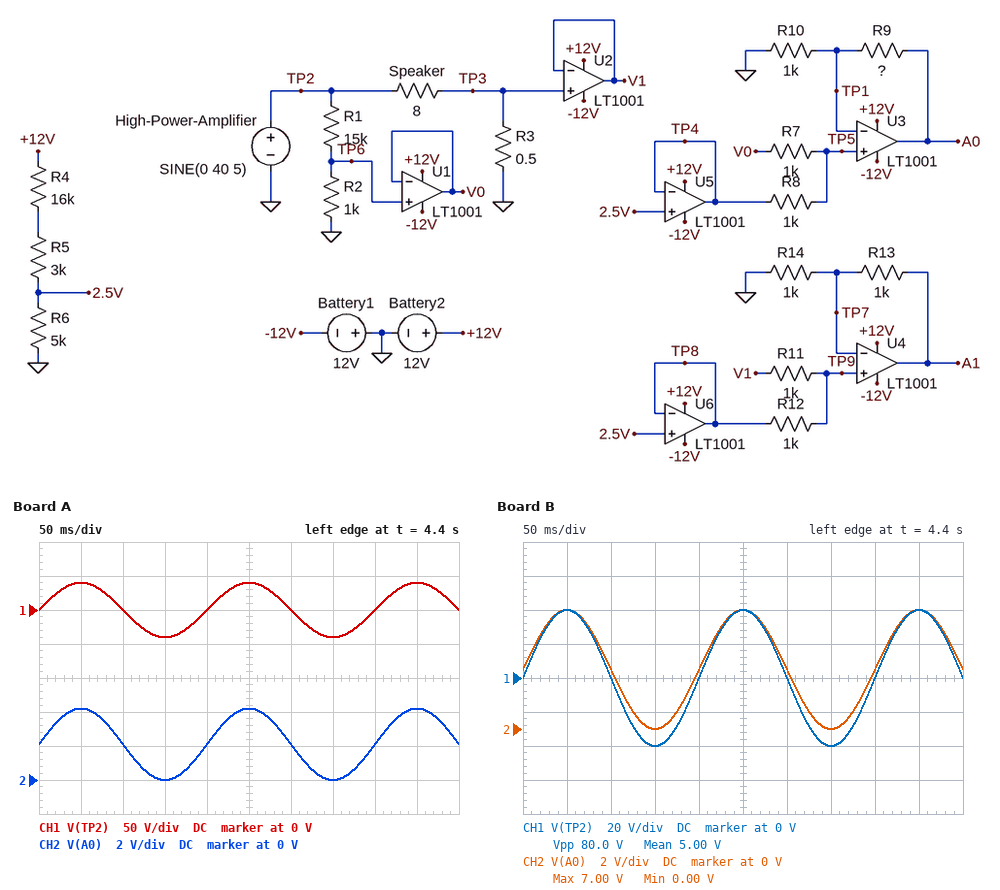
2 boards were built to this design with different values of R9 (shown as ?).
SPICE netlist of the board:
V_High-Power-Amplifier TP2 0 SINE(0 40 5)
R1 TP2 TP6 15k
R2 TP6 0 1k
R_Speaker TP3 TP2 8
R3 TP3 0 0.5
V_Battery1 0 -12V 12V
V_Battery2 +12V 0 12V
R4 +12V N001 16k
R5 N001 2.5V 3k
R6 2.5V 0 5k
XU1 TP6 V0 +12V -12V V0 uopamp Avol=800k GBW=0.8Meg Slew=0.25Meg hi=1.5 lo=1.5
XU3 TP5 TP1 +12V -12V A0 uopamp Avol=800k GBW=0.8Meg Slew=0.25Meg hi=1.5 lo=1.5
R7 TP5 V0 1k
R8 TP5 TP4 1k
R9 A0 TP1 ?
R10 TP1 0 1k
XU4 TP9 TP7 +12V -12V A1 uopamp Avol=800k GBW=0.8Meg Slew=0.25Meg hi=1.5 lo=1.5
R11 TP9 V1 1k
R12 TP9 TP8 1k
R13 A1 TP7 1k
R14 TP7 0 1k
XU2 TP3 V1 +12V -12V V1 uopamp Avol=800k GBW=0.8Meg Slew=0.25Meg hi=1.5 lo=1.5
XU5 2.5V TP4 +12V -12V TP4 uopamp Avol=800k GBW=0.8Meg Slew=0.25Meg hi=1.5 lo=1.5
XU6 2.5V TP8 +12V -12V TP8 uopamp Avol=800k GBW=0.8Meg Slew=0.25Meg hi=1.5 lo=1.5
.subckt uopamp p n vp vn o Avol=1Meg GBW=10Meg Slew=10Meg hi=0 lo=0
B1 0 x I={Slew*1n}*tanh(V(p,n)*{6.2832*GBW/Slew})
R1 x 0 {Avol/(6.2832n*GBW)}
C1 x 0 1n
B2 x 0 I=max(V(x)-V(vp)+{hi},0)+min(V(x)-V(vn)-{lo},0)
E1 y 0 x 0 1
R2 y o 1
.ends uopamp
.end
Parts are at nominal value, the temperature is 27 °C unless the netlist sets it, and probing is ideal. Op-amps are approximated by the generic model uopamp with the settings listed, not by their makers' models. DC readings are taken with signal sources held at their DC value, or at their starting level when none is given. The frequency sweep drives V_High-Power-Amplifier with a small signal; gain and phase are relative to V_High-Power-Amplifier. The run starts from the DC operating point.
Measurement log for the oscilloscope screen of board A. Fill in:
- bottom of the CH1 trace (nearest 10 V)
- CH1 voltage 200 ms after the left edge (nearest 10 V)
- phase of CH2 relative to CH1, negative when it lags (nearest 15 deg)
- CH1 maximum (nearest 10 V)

-40 V
0 V
0 deg
40 V
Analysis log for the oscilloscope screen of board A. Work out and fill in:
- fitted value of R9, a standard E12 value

680 Ω
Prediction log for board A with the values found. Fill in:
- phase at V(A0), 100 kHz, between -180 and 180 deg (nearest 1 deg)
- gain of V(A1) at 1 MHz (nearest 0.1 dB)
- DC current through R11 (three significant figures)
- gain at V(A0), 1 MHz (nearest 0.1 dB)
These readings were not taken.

-19 deg
-37.3 dB
1.25 mA
-37.0 dB
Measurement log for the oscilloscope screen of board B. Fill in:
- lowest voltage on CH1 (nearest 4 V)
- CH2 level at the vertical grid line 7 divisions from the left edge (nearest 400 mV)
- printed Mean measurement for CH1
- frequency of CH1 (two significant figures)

-40 V
0 V
5.00 V
5.0 Hz
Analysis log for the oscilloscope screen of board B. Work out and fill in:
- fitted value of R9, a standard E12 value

1.8 kΩ
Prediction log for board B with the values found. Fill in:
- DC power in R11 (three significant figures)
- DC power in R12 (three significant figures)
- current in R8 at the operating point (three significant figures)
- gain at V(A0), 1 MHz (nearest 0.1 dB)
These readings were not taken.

1.56 mW
1.56 mW
1.25 mA
-36.5 dB
